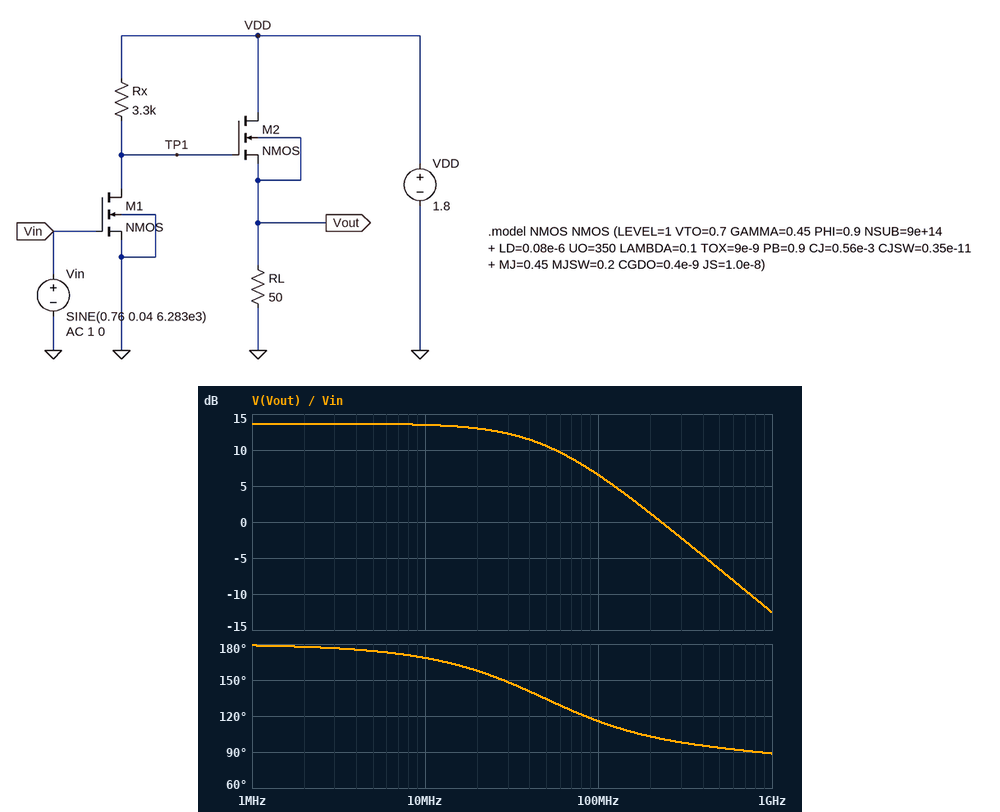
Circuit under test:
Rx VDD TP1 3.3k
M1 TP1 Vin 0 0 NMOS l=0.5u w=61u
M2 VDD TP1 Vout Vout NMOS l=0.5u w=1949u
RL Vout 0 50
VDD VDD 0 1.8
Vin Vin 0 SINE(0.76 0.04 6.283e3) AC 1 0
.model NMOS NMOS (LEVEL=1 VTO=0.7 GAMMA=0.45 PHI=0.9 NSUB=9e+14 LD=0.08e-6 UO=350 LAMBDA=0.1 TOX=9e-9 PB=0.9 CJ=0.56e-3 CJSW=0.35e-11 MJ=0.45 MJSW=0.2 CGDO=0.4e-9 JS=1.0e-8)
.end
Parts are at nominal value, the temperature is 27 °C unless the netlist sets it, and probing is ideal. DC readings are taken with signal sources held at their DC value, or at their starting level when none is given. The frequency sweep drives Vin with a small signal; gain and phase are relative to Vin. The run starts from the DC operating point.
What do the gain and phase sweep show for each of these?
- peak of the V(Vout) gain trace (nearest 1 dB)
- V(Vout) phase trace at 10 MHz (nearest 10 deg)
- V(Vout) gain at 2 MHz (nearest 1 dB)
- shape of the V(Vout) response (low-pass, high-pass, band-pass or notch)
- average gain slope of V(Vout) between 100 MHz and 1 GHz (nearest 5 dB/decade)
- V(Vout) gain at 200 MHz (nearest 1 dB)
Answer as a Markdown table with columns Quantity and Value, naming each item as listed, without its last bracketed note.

| Quantity | Value |
|---|---|
| peak of the V(Vout) gain trace | 14 dB |
| V(Vout) phase trace at 10 MHz | 170 deg |
| V(Vout) gain at 2 MHz | 14 dB |
| shape of the V(Vout) response | low-pass |
| average gain slope of V(Vout) between 100 MHz and 1 GHz | -20 dB/decade |
| V(Vout) gain at 200 MHz | 1 dB |
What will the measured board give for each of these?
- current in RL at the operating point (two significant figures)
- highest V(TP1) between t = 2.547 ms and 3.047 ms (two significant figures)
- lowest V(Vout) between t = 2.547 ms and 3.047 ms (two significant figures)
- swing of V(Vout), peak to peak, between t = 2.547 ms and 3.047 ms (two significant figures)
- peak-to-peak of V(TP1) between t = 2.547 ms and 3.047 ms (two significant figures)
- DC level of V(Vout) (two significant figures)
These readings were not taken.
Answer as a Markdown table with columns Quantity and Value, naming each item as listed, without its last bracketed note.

| Quantity | Value |
|---|---|
| current in RL at the operating point | 15 mA |
| highest V(TP1) between t = 2.547 ms and 3.047 ms | 1.8 V |
| lowest V(Vout) between t = 2.547 ms and 3.047 ms | 500 mV |
| swing of V(Vout), peak to peak, between t = 2.547 ms and 3.047 ms | 380 mV |
| peak-to-peak of V(TP1) between t = 2.547 ms and 3.047 ms | 430 mV |
| DC level of V(Vout) | 750 mV |
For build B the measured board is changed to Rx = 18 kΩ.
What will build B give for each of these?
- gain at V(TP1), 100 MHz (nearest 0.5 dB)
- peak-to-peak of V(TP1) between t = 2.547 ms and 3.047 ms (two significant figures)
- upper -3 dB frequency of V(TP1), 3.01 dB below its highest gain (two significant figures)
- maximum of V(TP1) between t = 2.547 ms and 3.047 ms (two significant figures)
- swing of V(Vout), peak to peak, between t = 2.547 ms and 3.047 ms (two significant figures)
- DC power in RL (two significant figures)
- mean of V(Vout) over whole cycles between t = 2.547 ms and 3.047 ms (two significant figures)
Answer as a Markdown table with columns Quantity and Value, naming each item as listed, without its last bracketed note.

| Quantity | Value |
|---|---|
| gain at V(TP1), 100 MHz | 6.5 dB |
| peak-to-peak of V(TP1) between t = 2.547 ms and 3.047 ms | 1.6 V |
| upper -3 dB frequency of V(TP1), 3.01 dB below its highest gain | 8.2 MHz |
| maximum of V(TP1) between t = 2.547 ms and 3.047 ms | 1.7 V |
| swing of V(Vout), peak to peak, between t = 2.547 ms and 3.047 ms | 800 mV |
| DC power in RL | 520 µW |
| mean of V(Vout) over whole cycles between t = 2.547 ms and 3.047 ms | 310 mV |
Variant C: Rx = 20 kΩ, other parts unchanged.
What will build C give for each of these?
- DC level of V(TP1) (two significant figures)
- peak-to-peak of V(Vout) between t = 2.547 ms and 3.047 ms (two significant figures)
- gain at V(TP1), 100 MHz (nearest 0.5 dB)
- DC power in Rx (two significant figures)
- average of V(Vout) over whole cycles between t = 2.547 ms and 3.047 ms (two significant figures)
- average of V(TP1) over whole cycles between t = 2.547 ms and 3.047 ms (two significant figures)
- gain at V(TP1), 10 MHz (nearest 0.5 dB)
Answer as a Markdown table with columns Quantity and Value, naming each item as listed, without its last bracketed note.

| Quantity | Value |
|---|---|
| DC level of V(TP1) | 860 mV |
| peak-to-peak of V(Vout) between t = 2.547 ms and 3.047 ms | 790 mV |
| gain at V(TP1), 100 MHz | 6.0 dB |
| DC power in Rx | 44 µW |
| average of V(Vout) over whole cycles between t = 2.547 ms and 3.047 ms | 290 mV |
| average of V(TP1) over whole cycles between t = 2.547 ms and 3.047 ms | 830 mV |
| gain at V(TP1), 10 MHz | 24.5 dB |
